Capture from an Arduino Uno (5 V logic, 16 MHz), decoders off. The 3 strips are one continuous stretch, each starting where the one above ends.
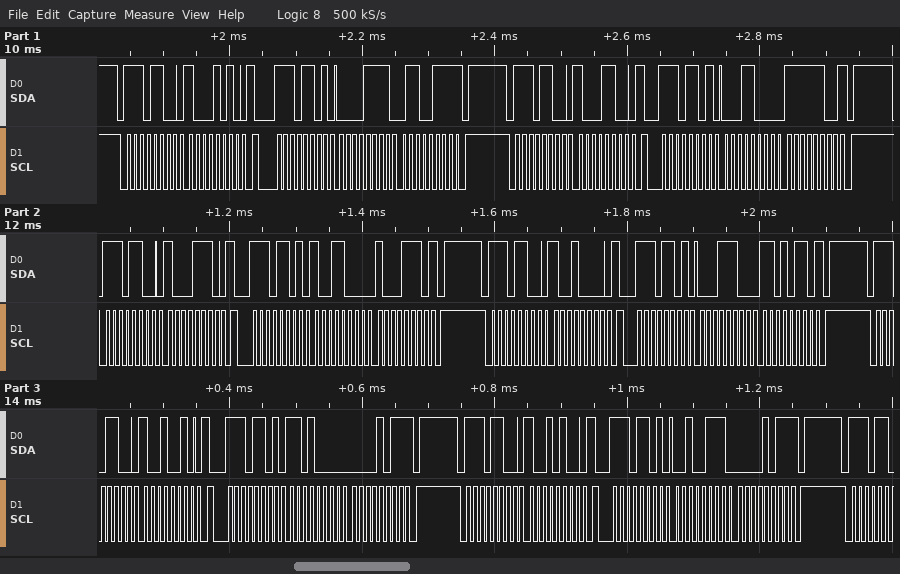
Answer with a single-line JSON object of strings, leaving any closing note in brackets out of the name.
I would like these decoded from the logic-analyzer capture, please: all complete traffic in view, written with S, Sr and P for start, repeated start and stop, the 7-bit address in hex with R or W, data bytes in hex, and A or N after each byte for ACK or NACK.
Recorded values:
{"all complete traffic in view, written with S, Sr and P for start, repeated start and stop, the 7-bit address in hex with R or W, data bytes in hex, and A or N after each byte for ACK or NACK": "S 76W A 8A A Sr 76R A 0F A 67 N P S 76W A 8C A Sr 76R A 18 A FC N P S 76W A 8E A Sr 76R A 98 A 8E N P S 76W A 90 A Sr 76R A 1C A D6 N P S 76W A 92 A Sr 76R A D0 A 0B N P S 76W A 94 A Sr 76R A 27 A 0B N P"}
